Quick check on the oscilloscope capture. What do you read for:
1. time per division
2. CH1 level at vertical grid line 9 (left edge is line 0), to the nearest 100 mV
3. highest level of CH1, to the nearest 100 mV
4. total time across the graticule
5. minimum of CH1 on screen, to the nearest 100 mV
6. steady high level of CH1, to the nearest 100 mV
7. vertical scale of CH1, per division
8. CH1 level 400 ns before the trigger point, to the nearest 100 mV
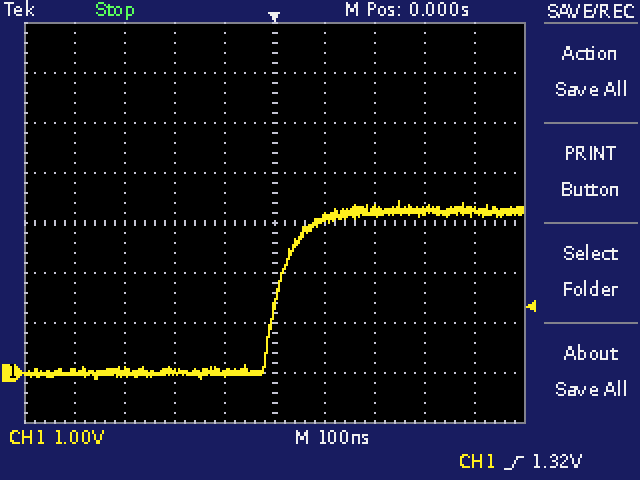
100 ns
3.2 V
3.4 V
1 µs
-100 mV
3.2 V
1 V
0.0 V
